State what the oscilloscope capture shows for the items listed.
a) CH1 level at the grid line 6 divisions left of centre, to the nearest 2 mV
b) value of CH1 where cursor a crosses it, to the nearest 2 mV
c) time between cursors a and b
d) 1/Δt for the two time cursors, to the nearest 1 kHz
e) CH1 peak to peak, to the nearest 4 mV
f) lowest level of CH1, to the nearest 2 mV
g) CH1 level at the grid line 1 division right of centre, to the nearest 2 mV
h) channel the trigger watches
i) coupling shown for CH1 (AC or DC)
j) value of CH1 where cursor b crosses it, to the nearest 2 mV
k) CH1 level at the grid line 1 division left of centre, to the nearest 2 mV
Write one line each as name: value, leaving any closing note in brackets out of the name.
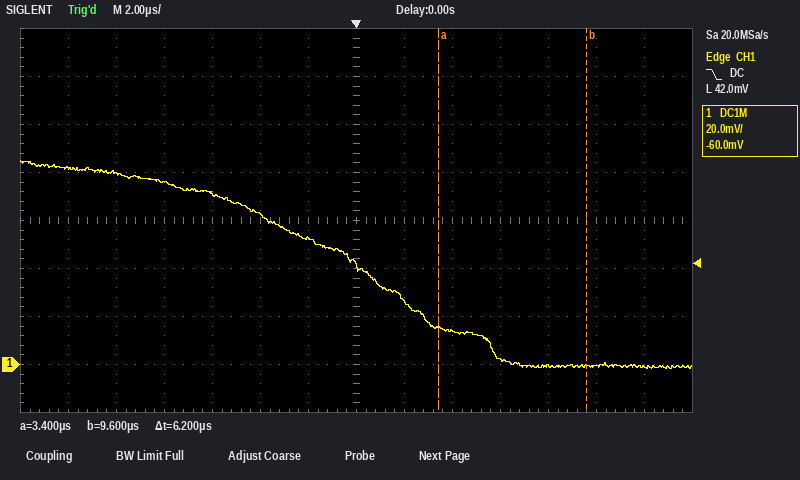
CH1 level at the grid line 6 divisions left of centre, to the nearest 2 mV: 82 mV
value of CH1 where cursor a crosses it, to the nearest 2 mV: 16 mV
time between cursors a and b: 6.2 µs
1/Δt for the two time cursors, to the nearest 1 kHz: 161 kHz
CH1 peak to peak, to the nearest 4 mV: 88 mV
lowest level of CH1, to the nearest 2 mV: -2 mV
CH1 level at the grid line 1 division right of centre, to the nearest 2 mV: 26 mV
channel the trigger watches: CH1
coupling shown for CH1: DC
value of CH1 where cursor b crosses it, to the nearest 2 mV: 0 mV
CH1 level at the grid line 1 division left of centre, to the nearest 2 mV: 52 mV
